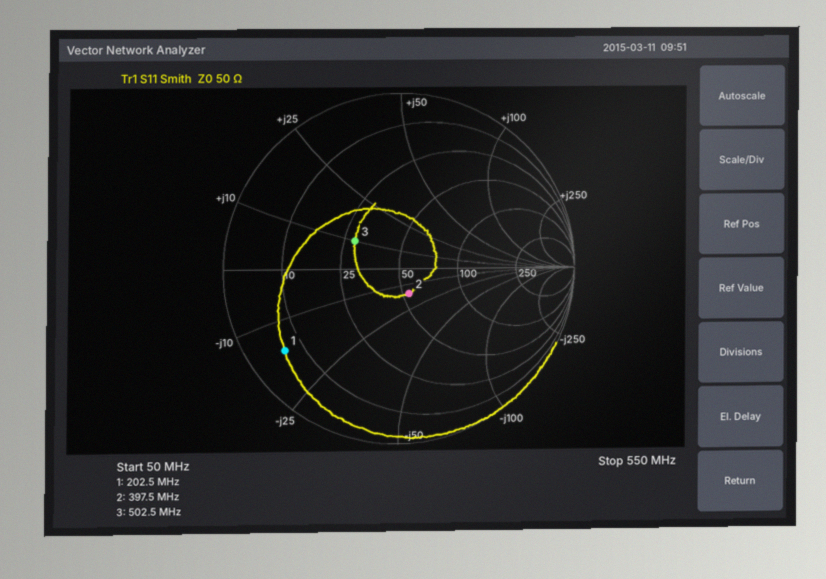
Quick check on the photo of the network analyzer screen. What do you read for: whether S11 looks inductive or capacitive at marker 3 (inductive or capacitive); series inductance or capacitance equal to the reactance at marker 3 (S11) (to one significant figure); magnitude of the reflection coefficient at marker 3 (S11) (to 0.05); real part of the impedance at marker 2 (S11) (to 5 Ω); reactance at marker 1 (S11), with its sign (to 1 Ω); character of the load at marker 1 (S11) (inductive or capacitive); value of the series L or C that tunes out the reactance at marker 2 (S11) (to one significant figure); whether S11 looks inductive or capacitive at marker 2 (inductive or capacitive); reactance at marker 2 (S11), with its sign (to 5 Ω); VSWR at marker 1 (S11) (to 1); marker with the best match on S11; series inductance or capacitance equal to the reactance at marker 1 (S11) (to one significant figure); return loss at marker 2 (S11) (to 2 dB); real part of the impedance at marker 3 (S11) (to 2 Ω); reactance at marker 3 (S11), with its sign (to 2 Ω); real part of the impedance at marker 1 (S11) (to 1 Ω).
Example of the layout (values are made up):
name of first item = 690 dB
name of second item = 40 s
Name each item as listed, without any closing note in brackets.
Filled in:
whether S11 looks inductive or capacitive at marker 3 = inductive
series inductance or capacitance equal to the reactance at marker 3 (S11) = 3 nH
magnitude of the reflection coefficient at marker 3 (S11) = 0.30
real part of the impedance at marker 2 (S11) = 55 Ω
reactance at marker 1 (S11), with its sign = -16 Ω
character of the load at marker 1 (S11) = capacitive
value of the series L or C that tunes out the reactance at marker 2 (S11) = 6 nH
whether S11 looks inductive or capacitive at marker 2 = capacitive
reactance at marker 2 (S11), with its sign = -15 Ω
VSWR at marker 1 (S11) = 9
marker with the best match on S11 = marker 2
series inductance or capacitance equal to the reactance at marker 1 (S11) = 50 pF
return loss at marker 2 (S11) = 16 dB
real part of the impedance at marker 3 (S11) = 28 Ω
reactance at marker 3 (S11), with its sign = +10 Ω
real part of the impedance at marker 1 (S11) = 6 Ω
